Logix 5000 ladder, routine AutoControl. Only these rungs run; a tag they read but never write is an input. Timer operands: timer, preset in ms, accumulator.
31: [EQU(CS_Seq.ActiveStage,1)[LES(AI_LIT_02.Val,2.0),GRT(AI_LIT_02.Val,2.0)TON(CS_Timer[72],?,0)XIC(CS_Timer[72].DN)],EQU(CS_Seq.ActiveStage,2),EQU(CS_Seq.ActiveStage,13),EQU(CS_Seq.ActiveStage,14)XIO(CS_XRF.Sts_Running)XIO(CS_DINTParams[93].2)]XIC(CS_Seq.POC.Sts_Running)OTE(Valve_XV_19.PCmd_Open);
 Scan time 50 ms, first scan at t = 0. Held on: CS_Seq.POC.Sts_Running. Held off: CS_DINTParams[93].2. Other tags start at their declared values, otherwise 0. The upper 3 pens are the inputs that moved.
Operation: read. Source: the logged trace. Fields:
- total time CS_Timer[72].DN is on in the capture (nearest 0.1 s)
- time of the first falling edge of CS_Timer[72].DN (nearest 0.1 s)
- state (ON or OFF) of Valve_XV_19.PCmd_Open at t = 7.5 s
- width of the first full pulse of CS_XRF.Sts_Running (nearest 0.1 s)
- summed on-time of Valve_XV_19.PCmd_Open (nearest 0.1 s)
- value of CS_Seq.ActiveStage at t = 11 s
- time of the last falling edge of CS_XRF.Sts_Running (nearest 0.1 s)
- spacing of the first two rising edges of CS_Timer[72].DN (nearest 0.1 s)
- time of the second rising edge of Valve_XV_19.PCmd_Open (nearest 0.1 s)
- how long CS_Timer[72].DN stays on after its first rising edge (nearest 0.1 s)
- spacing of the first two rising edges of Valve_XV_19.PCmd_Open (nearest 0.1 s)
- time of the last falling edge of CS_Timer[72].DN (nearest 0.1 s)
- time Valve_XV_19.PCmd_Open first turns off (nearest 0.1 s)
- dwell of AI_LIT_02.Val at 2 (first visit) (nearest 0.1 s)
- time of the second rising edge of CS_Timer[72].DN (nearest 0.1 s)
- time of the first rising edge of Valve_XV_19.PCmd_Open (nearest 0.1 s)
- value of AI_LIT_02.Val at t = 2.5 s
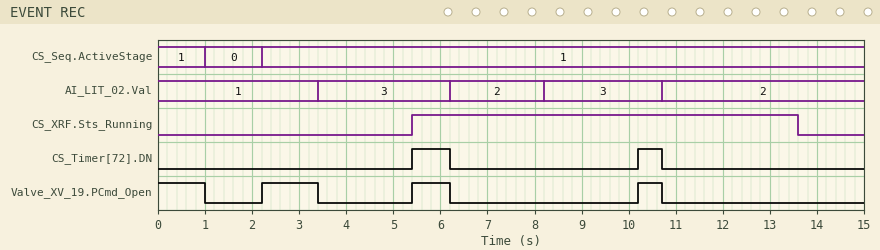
1.3 s
6.2 s
OFF
8.2 s
3.5 s
1
13.6 s
4.8 s
5.4 s
0.8 s
3.2 s
10.7 s
1.0 s
2.0 s
10.2 s
2.2 s
1
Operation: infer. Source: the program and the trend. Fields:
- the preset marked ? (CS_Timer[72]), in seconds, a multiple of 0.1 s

2.0 s
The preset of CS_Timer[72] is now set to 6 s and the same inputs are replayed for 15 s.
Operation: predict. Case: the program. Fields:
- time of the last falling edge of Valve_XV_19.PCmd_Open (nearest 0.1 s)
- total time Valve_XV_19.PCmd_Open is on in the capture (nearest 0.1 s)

3.4 s
2.2 s
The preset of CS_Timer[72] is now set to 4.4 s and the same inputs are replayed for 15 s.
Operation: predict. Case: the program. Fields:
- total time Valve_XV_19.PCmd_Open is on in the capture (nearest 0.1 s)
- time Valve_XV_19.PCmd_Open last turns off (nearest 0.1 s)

2.2 s
3.4 s
